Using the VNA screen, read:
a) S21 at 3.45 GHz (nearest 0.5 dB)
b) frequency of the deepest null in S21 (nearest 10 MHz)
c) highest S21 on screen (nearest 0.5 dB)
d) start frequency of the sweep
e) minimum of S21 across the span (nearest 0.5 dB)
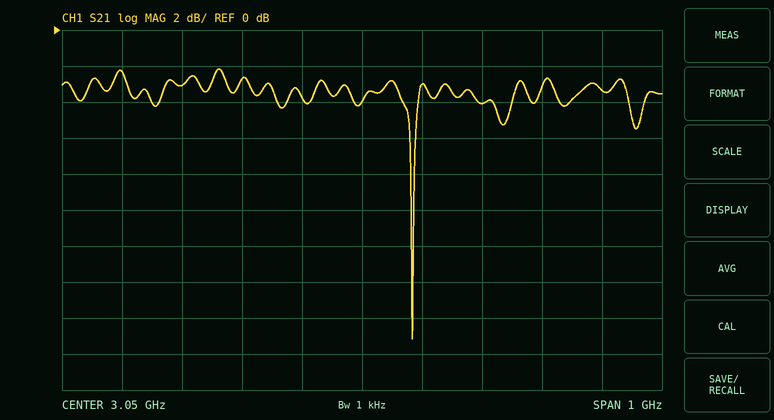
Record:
-3.5 dB
3.13 GHz
-2.0 dB
2.55 GHz
-17.0 dB
